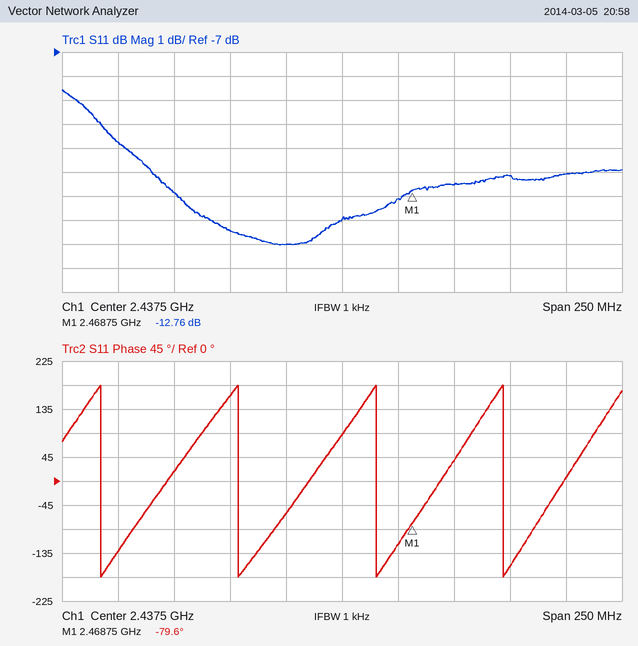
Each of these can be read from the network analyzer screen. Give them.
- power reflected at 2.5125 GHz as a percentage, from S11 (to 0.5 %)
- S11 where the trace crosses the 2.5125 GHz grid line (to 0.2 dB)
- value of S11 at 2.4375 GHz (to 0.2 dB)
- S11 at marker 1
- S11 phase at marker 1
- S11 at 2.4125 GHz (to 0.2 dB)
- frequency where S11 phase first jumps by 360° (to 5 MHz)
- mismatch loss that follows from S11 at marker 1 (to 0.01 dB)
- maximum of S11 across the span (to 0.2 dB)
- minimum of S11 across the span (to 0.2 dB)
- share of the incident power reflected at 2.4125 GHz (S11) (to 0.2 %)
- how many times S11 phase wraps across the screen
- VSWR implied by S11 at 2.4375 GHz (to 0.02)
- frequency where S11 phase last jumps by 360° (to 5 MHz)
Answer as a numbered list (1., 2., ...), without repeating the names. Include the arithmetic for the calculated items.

1. 10^(-12.2/10) ≈ 6.0 %
2. -12.2 dB
3. -14.0 dB
4. -12.76 dB
5. -79.6°
6. -15.0 dB
7. 2.330 GHz
8. −10 log10(1 − 10^(-12.76/10)) ≈ 0.24 dB
9. -8.6 dB
10. -15.0 dB
11. 10^(-15/10) ≈ 3.2 %
12. 4
13. |Γ| = 10^(-14/20) = 0.1995; VSWR = (1 + 0.1995)/(1 − 0.1995) ≈ 1.50
14. 2.510 GHz
